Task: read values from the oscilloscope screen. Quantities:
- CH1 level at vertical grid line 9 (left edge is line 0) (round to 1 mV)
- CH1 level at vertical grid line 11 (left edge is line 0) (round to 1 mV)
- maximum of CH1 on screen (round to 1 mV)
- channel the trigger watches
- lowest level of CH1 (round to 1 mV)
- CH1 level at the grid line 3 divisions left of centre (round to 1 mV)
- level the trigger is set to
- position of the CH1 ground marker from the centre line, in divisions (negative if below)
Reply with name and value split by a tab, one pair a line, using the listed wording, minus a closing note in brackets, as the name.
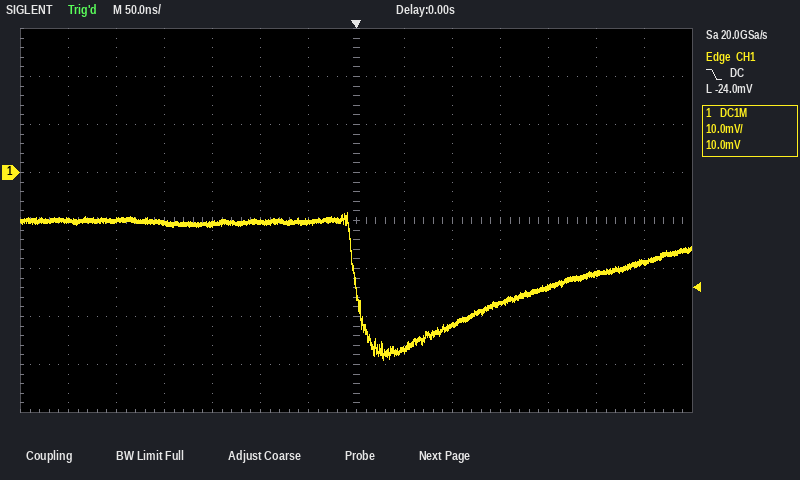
CH1 level at vertical grid line 9 (left edge is line 0)	-32 mV
CH1 level at vertical grid line 11 (left edge is line 0)	-24 mV
maximum of CH1 on screen	-8 mV
channel the trigger watches	CH1
lowest level of CH1	-39 mV
CH1 level at the grid line 3 divisions left of centre	-11 mV
level the trigger is set to	-24.0 mV
position of the CH1 ground marker from the centre line, in divisions	+1.0 div
